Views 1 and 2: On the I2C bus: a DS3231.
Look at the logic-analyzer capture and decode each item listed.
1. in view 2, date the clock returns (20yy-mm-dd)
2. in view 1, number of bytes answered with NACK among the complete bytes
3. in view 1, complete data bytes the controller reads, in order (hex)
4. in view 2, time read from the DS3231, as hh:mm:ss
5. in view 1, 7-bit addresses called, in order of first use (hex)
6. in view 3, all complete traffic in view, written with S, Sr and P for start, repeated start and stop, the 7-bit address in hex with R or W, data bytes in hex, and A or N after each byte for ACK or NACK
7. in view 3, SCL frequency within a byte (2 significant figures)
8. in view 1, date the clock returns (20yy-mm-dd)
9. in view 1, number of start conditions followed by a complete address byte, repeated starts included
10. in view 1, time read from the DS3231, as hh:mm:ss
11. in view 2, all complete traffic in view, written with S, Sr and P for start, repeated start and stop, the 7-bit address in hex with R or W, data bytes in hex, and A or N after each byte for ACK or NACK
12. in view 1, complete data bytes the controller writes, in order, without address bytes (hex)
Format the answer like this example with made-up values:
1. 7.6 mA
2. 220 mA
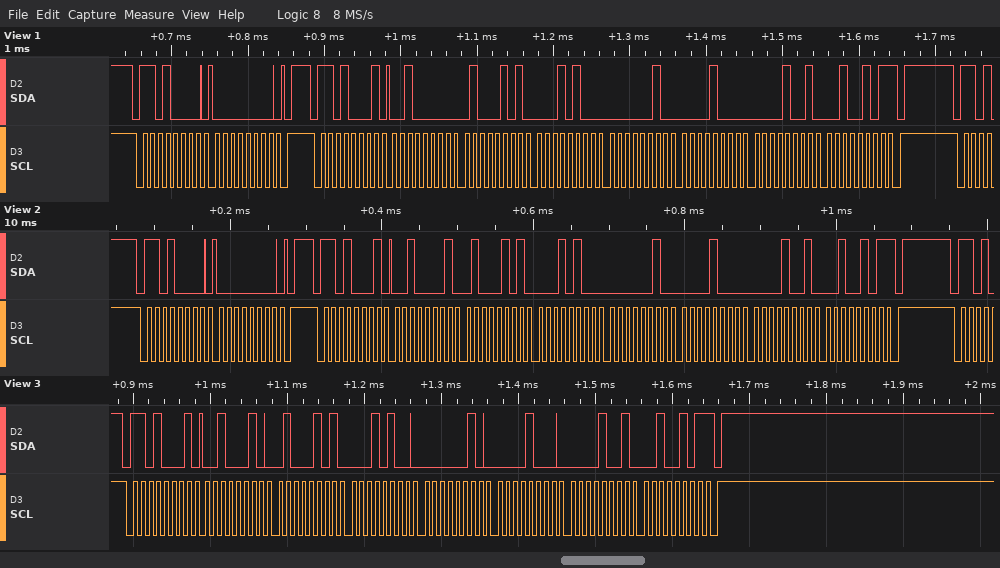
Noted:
1. 2025-09-08
2. 1
3. 20 45 14 02 08 09 25
4. 14:45:21
5. 0x68
6. S 68R A 22 A 45 A 14 A 02 A 08 A 09 A 25 N P
7. 100 kHz
8. 2025-09-08
9. 2
10. 14:45:20
11. S 68W A 00 A P S 68R A 21 A 45 A 14 A 02 A 08 A 09 A 25 N P
12. 00
